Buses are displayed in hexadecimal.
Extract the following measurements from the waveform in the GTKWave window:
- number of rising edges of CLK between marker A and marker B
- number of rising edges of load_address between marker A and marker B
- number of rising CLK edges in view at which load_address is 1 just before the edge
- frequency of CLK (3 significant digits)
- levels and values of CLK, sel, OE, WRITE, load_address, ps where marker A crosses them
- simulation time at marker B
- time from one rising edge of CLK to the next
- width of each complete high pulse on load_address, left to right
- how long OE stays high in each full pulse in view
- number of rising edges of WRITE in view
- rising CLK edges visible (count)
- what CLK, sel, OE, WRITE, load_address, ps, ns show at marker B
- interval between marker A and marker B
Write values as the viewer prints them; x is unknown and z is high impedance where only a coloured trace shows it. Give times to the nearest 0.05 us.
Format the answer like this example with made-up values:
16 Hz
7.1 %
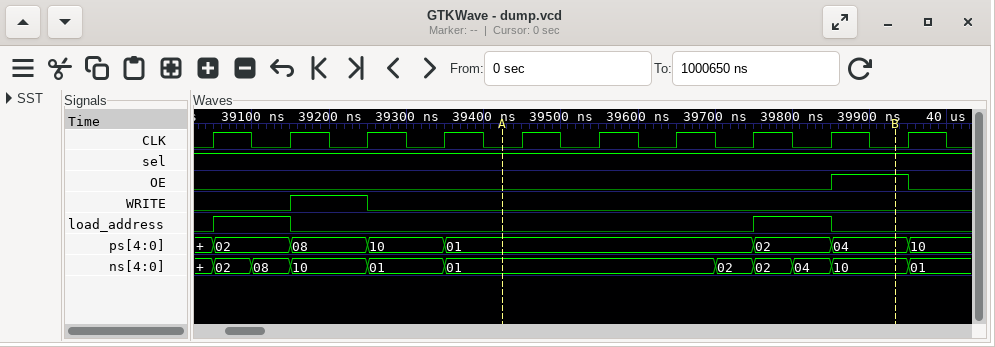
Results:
5
1
2
10.0 MHz
CLK=0, sel=1, OE=0, WRITE=0, load_address=0, ps=01
39.95 us
0.1 us
0.1 us, 0.1 us
0.1 us
1
10
CLK=0, sel=1, OE=1, WRITE=0, load_address=0, ps=04, ns=10
0.5 us
